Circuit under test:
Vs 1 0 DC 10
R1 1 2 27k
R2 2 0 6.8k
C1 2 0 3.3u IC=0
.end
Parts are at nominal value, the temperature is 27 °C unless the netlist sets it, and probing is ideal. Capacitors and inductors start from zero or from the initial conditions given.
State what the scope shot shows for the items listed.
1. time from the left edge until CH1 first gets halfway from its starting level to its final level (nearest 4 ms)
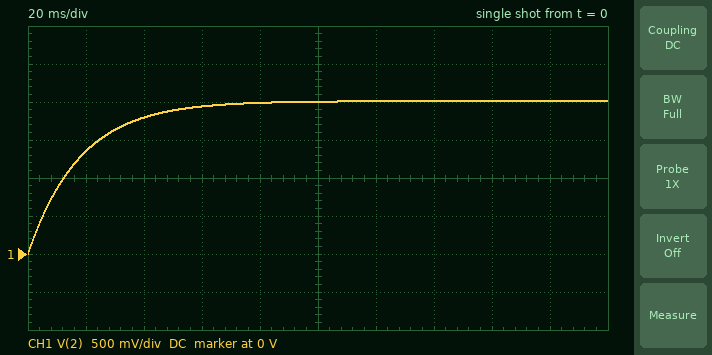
12 ms
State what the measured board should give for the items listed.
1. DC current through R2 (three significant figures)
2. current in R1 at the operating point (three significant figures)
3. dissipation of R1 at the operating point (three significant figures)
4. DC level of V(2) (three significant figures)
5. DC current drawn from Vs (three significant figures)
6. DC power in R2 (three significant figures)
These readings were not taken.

296 µA
296 µA
2.36 mW
2.01 V
296 µA
595 µW
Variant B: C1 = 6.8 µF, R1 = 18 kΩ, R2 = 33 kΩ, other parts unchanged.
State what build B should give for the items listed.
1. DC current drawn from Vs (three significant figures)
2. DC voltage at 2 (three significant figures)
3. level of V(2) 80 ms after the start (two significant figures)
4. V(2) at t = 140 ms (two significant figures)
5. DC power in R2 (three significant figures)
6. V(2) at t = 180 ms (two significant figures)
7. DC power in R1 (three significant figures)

196 µA
6.47 V
4.1 V
5.4 V
1.27 mW
5.8 V
692 µW
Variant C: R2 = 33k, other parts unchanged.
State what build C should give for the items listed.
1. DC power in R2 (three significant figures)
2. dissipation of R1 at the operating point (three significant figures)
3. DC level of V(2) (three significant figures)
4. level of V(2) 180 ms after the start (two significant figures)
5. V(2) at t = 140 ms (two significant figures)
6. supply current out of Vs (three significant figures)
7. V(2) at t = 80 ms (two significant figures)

917 µW
750 µW
5.50 V
5.4 V
5.2 V
167 µA
4.4 V
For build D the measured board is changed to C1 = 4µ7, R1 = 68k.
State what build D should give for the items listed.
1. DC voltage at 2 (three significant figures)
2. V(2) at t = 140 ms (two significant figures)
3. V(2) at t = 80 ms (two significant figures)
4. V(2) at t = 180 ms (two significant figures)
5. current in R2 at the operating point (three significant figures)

909 mV
900 mV
850 mV
910 mV
134 µA
